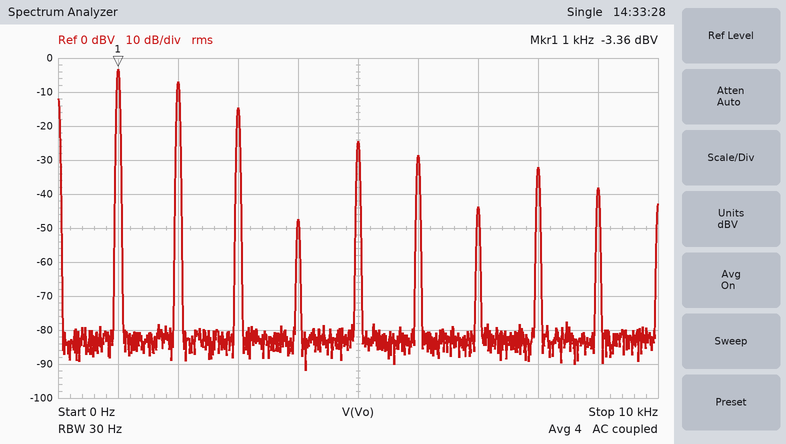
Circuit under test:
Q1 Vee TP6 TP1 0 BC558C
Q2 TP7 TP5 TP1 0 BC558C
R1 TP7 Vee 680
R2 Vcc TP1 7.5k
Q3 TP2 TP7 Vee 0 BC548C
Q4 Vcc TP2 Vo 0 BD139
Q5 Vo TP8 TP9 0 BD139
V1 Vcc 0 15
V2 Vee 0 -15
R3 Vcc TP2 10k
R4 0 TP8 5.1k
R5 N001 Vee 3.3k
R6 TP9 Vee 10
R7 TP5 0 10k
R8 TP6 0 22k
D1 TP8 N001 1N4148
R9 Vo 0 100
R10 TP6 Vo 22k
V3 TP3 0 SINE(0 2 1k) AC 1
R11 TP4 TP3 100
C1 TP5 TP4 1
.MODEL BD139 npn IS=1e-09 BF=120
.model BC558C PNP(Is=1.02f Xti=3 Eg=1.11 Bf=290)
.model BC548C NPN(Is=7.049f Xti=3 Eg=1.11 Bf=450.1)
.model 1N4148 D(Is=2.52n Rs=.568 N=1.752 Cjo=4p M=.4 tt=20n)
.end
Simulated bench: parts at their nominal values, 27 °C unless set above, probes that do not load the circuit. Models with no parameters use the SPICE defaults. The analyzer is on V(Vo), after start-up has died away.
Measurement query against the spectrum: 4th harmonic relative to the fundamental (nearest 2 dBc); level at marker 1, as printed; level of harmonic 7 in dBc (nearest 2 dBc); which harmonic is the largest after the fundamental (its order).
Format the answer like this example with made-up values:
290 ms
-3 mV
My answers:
-44 dBc
-3.36 dBV
-40 dBc
2
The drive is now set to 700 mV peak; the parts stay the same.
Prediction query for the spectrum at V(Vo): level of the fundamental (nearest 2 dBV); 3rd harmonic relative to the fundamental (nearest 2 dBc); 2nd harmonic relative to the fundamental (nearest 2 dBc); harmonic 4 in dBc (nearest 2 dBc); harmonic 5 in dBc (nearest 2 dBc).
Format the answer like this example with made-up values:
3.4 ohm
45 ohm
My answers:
-132 dBV
-2 dBc
0 dBc
-2 dBc
-4 dBc
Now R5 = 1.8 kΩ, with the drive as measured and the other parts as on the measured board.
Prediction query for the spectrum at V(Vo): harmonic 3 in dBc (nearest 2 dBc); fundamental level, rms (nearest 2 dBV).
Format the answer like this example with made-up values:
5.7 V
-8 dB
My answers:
-32 dBc
2 dBV
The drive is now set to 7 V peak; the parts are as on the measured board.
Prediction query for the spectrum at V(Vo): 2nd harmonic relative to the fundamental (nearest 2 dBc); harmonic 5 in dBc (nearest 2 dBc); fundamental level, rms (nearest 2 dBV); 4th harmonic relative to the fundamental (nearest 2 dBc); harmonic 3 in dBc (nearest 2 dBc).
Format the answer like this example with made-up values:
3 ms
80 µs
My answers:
-6 dBc
-28 dBc
12 dBV
-20 dBc
-26 dBc
